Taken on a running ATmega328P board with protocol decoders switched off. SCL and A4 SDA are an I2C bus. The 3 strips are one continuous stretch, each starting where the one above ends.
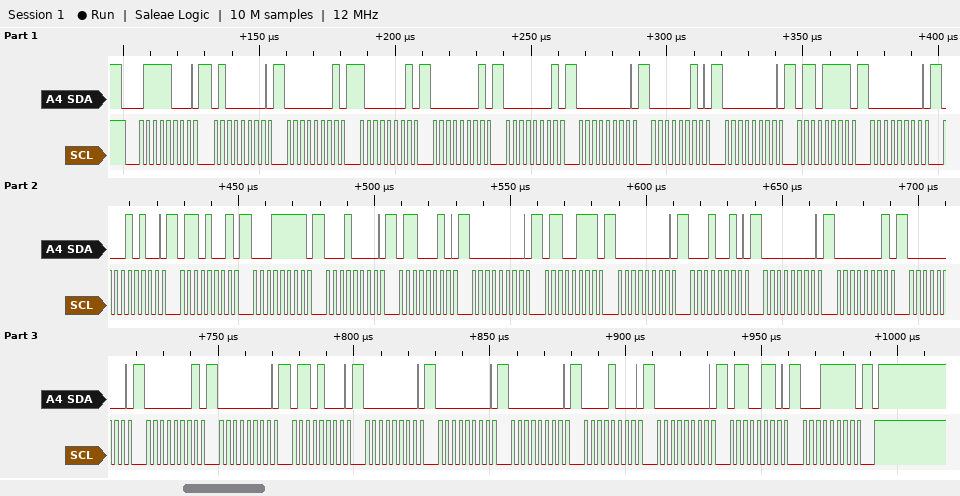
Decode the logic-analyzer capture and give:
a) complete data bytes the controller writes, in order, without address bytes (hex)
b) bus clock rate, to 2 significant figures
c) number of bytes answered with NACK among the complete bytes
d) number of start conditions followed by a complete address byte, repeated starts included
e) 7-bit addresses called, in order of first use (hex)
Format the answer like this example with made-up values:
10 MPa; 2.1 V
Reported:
40 01 81 01 01 00 02 00 6F 00 14 69 1F 10 62 00 67 00 12 00 01 00 01 00 68 00 00 00 08 00 66 1F; 400 kHz; 0; 1; 0x3C
